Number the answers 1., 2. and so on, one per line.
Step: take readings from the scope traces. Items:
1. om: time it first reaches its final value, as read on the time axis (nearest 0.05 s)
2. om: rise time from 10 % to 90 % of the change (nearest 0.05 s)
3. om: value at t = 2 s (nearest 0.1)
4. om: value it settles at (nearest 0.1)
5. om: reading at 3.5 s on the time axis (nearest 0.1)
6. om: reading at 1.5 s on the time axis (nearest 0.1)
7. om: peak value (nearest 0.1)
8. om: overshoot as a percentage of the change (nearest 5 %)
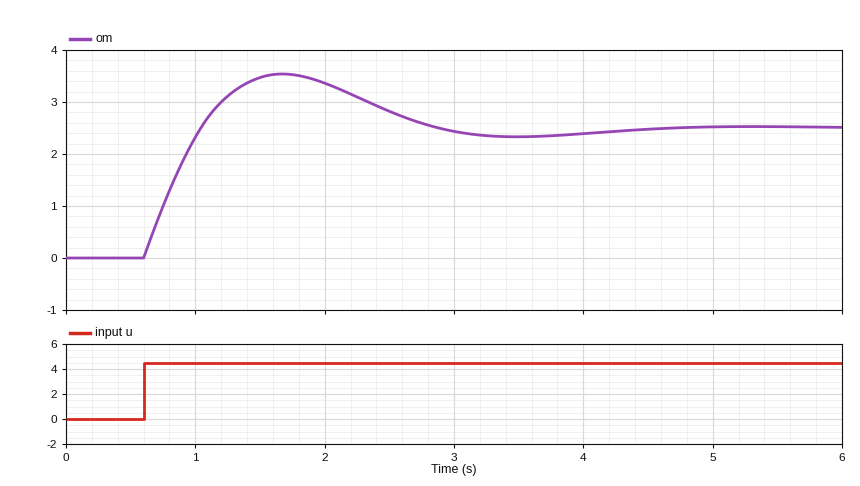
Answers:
1. 1.05 s
2. 0.35 s
3. 3.4
4. 2.5
5. 2.3
6. 3.5
7. 3.5
8. 40 %
